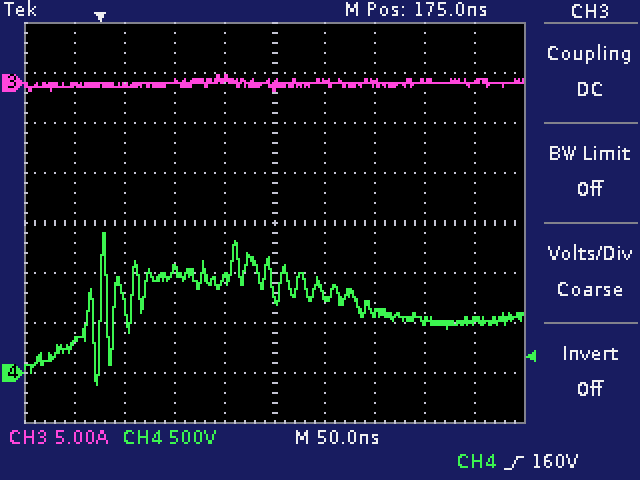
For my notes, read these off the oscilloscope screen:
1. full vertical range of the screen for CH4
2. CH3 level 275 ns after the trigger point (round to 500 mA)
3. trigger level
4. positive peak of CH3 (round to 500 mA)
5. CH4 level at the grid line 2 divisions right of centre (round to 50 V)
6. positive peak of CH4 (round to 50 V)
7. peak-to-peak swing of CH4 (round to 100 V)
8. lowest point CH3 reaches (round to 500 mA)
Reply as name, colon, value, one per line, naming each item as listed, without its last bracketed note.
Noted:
full vertical range of the screen for CH4: 4 kV
CH3 level 275 ns after the trigger point: 0.0 A
trigger level: 160 V
positive peak of CH3: 1.0 A
CH4 level at the grid line 2 divisions right of centre: 600 V
positive peak of CH4: 1.40 kV
peak-to-peak swing of CH4: 1.50 kV
lowest point CH3 reaches: -1.0 A
